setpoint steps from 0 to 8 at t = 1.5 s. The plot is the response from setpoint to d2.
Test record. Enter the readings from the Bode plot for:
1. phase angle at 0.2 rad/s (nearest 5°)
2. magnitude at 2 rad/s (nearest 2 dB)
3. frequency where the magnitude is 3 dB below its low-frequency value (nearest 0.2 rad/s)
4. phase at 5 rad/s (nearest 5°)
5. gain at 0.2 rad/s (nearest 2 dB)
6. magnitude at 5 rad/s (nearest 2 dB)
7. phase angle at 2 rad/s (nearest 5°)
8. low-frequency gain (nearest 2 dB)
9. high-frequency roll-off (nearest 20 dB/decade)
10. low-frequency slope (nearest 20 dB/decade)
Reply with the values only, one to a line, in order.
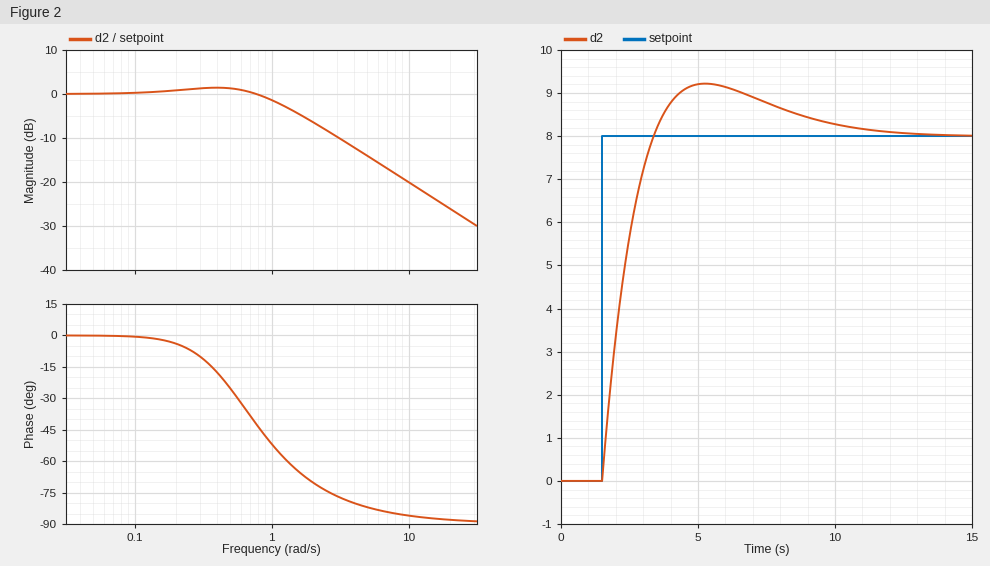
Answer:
-5°
-6 dB
1.2 rad/s
-80°
0 dB
-14 dB
-70°
0 dB
-20 dB/decade
0 dB/decade
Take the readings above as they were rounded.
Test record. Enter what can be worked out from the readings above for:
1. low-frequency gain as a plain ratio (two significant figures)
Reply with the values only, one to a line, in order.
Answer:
1.0
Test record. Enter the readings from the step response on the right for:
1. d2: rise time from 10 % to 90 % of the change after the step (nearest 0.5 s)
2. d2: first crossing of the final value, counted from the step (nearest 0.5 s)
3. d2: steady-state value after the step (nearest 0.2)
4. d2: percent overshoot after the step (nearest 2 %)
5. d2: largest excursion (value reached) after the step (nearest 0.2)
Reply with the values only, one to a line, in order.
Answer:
1.5 s
2.0 s
8.0
16 %
9.2
